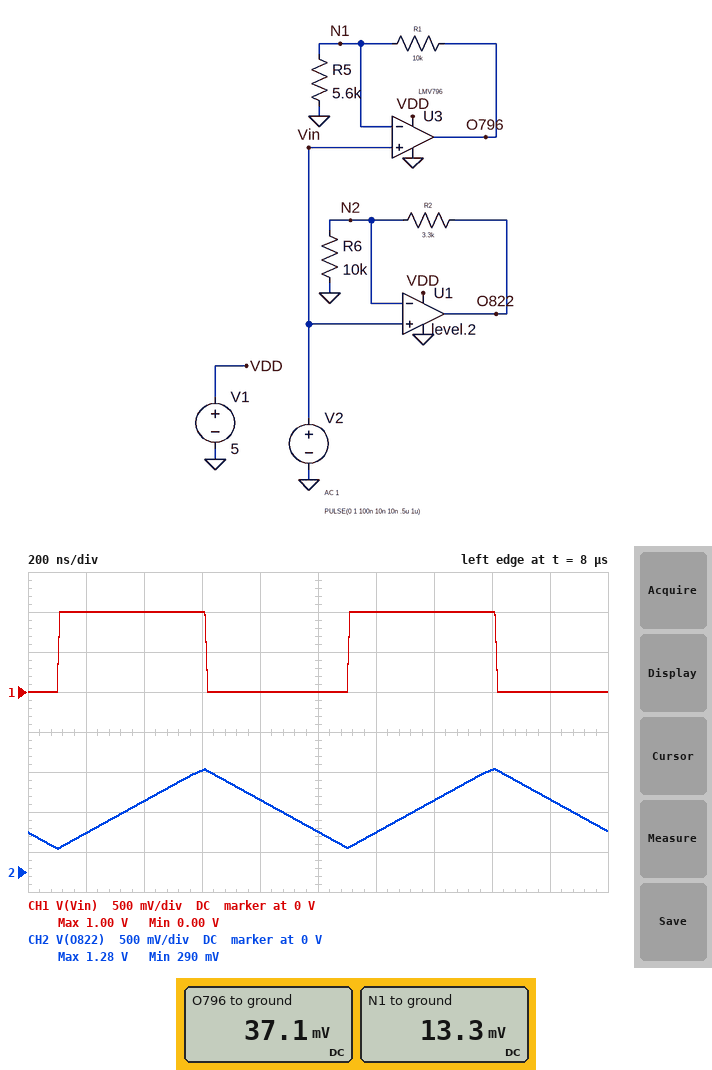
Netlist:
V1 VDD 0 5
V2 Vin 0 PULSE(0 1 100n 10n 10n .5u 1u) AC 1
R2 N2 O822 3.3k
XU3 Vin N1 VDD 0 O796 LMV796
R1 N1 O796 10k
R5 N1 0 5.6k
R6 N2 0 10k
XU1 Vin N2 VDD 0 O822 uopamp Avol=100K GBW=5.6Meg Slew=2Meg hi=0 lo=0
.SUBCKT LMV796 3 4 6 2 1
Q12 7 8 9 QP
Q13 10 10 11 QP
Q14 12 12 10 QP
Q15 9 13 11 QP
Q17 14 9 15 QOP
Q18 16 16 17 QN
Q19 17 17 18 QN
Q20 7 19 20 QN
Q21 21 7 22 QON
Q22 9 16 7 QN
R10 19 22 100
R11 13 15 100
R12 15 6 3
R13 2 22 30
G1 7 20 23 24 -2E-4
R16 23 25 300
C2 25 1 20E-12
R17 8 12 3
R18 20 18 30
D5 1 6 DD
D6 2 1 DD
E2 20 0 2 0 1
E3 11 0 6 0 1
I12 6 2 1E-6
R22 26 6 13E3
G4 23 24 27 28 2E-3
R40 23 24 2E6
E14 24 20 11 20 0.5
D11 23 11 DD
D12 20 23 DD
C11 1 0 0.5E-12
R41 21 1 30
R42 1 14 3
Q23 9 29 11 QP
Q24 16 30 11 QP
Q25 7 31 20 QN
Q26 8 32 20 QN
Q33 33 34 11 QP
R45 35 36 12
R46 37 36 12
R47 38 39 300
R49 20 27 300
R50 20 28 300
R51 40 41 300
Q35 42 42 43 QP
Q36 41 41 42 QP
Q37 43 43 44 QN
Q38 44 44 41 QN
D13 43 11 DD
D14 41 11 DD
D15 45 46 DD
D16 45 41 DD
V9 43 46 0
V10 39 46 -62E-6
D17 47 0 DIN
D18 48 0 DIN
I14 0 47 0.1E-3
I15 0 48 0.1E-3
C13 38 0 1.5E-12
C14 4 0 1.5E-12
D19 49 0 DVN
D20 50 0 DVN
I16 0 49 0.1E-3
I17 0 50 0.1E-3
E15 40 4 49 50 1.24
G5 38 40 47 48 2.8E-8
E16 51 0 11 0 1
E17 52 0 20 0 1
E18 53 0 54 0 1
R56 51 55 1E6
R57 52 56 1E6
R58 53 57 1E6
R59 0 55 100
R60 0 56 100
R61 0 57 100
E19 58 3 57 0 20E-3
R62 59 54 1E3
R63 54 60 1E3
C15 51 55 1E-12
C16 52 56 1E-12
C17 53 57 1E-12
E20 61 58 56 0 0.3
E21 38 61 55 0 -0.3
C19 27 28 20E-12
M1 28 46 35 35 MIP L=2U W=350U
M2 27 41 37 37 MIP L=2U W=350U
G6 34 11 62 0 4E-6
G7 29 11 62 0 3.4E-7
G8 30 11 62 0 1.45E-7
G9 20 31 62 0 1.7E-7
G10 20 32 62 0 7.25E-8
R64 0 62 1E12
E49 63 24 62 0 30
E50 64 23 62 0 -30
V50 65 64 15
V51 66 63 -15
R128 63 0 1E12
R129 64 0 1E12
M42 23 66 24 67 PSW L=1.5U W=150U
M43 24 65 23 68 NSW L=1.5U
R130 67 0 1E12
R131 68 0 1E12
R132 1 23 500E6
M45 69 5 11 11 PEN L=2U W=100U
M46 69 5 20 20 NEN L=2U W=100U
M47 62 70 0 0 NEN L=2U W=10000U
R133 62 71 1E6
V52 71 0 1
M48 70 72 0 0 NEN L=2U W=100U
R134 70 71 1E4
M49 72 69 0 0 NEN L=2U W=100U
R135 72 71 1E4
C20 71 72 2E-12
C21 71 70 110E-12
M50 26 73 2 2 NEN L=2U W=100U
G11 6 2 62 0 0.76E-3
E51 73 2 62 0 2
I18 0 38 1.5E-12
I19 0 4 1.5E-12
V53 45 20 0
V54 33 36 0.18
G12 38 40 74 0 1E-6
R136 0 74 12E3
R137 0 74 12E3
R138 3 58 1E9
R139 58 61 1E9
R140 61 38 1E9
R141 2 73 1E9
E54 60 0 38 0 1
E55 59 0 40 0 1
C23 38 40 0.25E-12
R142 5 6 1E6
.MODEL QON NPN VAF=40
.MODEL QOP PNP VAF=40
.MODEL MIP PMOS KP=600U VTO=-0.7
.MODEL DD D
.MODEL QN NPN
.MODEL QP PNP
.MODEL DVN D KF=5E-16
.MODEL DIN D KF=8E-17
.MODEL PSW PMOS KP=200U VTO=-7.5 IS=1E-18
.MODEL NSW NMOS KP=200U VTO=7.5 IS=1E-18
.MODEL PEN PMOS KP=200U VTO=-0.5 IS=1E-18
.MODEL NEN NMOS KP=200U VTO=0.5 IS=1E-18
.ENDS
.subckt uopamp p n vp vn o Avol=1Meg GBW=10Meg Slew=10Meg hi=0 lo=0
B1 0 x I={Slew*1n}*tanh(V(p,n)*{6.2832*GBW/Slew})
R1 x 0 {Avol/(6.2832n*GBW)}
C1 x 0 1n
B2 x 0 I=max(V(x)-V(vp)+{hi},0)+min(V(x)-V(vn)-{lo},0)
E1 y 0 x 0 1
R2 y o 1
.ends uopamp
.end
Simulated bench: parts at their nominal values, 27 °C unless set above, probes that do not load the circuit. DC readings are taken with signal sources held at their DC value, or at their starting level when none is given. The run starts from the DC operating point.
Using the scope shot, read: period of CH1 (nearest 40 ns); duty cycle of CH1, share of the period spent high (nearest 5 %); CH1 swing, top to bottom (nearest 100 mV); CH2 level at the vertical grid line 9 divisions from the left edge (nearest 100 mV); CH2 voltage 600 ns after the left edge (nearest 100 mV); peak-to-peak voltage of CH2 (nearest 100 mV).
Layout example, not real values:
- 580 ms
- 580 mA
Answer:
- 1.00 µs
- 50 %
- 1.0 V
- 900 mV
- 1.3 V
- 1.0 V
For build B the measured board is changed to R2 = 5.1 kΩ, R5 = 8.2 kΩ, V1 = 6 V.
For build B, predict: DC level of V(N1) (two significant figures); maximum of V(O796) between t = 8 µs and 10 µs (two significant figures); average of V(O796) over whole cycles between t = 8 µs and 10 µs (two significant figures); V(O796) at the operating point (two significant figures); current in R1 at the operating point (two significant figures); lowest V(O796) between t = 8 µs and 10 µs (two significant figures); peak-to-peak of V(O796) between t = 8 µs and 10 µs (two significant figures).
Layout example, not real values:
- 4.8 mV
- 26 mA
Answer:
- 18 mV
- 2.3 V
- 960 mV
- 40 mV
- 2.2 µA
- -78 mV
- 2.4 V
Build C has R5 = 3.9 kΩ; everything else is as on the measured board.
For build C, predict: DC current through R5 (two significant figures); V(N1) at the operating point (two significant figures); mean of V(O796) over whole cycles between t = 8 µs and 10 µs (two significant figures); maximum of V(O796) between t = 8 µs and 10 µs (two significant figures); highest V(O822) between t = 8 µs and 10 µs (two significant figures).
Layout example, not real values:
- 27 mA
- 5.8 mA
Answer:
- 2.7 µA
- 10 mV
- 1.7 V
- 3.6 V
- 1.3 V
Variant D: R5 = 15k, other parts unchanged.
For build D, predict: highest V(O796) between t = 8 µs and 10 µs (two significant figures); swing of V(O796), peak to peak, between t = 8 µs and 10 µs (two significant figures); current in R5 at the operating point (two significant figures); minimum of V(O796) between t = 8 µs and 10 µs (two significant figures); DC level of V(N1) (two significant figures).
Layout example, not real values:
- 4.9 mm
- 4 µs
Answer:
- 1.8 V
- 1.9 V
- 1.5 µA
- -80 mV
- 22 mV
